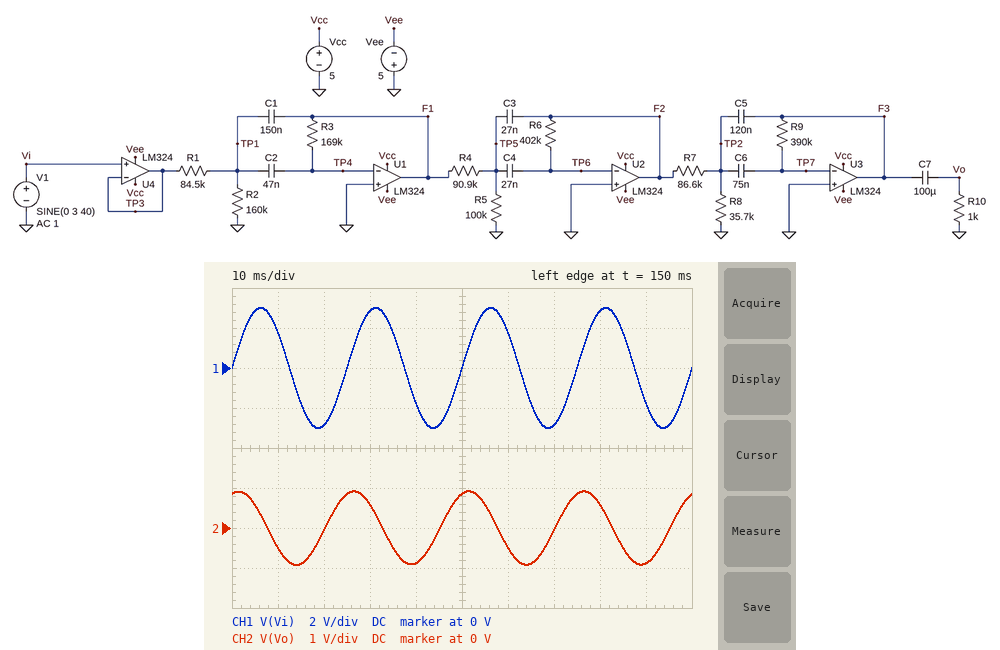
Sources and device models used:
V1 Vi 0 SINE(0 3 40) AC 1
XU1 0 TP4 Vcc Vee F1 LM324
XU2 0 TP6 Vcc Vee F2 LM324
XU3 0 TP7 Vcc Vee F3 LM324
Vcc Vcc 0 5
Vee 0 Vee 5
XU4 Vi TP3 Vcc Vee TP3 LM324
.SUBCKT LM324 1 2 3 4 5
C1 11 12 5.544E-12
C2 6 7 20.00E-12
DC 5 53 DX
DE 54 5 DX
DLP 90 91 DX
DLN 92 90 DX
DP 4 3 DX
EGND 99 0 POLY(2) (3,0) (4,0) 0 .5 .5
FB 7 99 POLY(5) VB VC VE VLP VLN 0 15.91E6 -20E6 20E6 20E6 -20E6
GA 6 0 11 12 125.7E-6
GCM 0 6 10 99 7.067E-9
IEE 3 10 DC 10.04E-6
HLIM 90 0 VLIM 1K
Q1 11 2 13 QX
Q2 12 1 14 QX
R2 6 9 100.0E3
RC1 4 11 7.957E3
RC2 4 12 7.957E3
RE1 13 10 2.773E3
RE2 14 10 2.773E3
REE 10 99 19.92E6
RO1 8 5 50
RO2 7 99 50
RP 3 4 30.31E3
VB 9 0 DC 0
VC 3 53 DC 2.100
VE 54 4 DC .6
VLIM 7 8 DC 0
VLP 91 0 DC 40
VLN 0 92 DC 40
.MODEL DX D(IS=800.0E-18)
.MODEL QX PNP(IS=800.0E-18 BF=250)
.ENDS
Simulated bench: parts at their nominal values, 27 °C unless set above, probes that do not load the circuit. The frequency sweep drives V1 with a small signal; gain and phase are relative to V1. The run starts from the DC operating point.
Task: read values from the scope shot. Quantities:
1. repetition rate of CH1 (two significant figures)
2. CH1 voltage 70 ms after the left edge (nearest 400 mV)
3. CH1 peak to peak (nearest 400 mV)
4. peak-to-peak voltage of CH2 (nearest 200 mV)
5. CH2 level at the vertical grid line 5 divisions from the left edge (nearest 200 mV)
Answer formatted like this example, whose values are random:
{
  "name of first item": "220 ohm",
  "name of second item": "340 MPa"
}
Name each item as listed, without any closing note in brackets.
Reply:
{
  "repetition rate of CH1": "40 Hz",
  "CH1 voltage 70 ms after the left edge": "-2.8 V",
  "CH1 peak to peak": "6.0 V",
  "peak-to-peak voltage of CH2": "1.8 V",
  "CH2 level at the vertical grid line 5 divisions from the left edge": "800 mV"
}
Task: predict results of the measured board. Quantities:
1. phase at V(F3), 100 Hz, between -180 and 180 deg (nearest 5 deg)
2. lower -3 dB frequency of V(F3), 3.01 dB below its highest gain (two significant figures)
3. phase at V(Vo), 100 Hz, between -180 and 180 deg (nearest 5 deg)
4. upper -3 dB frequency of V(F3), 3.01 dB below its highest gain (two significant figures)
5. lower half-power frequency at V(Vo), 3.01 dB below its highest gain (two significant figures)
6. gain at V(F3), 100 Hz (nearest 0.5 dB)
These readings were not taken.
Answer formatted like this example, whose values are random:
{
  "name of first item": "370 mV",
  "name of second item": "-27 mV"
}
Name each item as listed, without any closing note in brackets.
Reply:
{
  "phase at V(F3), 100 Hz, between -180 and 180 deg": "-50 deg",
  "lower -3 dB frequency of V(F3), 3.01 dB below its highest gain": "15 Hz",
  "phase at V(Vo), 100 Hz, between -180 and 180 deg": "-50 deg",
  "upper -3 dB frequency of V(F3), 3.01 dB below its highest gain": "30 Hz",
  "lower half-power frequency at V(Vo), 3.01 dB below its highest gain": "15 Hz",
  "gain at V(F3), 100 Hz": "-36.5 dB"
}
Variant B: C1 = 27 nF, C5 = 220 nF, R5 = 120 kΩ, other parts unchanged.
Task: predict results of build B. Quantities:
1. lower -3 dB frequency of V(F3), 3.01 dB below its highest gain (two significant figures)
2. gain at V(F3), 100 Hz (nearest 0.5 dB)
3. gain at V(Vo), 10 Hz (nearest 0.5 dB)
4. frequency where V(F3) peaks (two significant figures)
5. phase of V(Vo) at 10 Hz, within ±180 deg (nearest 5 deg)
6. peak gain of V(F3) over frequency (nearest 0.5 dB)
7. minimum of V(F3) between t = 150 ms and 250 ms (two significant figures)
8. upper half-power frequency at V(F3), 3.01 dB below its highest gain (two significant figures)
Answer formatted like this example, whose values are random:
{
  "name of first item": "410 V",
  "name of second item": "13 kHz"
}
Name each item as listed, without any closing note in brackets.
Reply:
{
  "lower -3 dB frequency of V(F3), 3.01 dB below its highest gain": "25 Hz",
  "gain at V(F3), 100 Hz": "-27.0 dB",
  "gain at V(Vo), 10 Hz": "-18.5 dB",
  "frequency where V(F3) peaks": "37 Hz",
  "phase of V(Vo) at 10 Hz, within ±180 deg": "20 deg",
  "peak gain of V(F3) over frequency": "-4.0 dB",
  "minimum of V(F3) between t = 150 ms and 250 ms": "-1.1 V",
  "upper half-power frequency at V(F3), 3.01 dB below its highest gain": "49 Hz"
}
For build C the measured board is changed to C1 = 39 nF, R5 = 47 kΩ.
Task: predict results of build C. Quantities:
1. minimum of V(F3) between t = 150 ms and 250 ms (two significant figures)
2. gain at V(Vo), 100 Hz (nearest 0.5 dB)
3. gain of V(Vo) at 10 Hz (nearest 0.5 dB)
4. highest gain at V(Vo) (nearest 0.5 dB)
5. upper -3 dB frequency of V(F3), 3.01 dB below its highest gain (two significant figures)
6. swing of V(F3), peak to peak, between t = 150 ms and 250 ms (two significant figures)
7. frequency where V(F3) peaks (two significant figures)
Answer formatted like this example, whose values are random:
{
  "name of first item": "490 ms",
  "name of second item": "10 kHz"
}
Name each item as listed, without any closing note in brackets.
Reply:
{
  "minimum of V(F3) between t = 150 ms and 250 ms": "-2.0 V",
  "gain at V(Vo), 100 Hz": "-23.5 dB",
  "gain of V(Vo) at 10 Hz": "-24.5 dB",
  "highest gain at V(Vo)": "-2.0 dB",
  "upper -3 dB frequency of V(F3), 3.01 dB below its highest gain": "57 Hz",
  "swing of V(F3), peak to peak, between t = 150 ms and 250 ms": "4.1 V",
  "frequency where V(F3) peaks": "44 Hz"
}
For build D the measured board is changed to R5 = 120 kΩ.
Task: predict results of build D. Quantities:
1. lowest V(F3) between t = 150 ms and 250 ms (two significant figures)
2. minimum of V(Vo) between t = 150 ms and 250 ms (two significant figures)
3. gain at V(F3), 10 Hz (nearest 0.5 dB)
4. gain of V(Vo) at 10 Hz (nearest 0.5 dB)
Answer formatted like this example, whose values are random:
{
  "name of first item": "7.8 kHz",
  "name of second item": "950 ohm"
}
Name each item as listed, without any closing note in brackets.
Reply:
{
  "lowest V(F3) between t = 150 ms and 250 ms": "-950 mV",
  "minimum of V(Vo) between t = 150 ms and 250 ms": "-940 mV",
  "gain at V(F3), 10 Hz": "-20.0 dB",
  "gain of V(Vo) at 10 Hz": "-20.5 dB"
}
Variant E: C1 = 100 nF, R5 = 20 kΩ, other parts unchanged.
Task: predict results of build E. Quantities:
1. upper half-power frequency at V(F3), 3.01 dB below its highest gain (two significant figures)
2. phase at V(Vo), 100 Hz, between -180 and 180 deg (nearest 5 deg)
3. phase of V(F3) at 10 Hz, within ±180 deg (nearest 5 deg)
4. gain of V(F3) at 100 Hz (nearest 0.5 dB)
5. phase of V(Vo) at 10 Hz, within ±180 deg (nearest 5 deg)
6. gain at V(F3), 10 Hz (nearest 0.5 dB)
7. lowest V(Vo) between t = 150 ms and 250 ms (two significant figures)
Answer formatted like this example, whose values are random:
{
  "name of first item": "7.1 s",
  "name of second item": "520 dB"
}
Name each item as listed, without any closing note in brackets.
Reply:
{
  "upper half-power frequency at V(F3), 3.01 dB below its highest gain": "33 Hz",
  "phase at V(Vo), 100 Hz, between -180 and 180 deg": "-35 deg",
  "phase of V(F3) at 10 Hz, within ±180 deg": "30 deg",
  "gain of V(F3) at 100 Hz": "-29.0 dB",
  "phase of V(Vo) at 10 Hz, within ±180 deg": "40 deg",
  "gain at V(F3), 10 Hz": "-30.0 dB",
  "lowest V(Vo) between t = 150 ms and 250 ms": "-440 mV"
}
